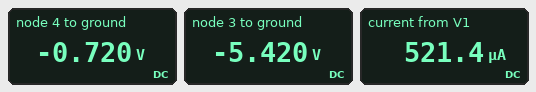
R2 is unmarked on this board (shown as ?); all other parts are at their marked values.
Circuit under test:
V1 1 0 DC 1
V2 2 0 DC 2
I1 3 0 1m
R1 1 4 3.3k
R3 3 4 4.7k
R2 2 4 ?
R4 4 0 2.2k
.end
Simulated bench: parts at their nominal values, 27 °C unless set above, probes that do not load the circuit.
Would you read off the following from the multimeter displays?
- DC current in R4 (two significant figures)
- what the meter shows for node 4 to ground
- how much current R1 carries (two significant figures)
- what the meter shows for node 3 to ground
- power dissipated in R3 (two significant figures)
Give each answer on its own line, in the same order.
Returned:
330 µA
-0.720 V
520 µA
-5.420 V
4.7 mW
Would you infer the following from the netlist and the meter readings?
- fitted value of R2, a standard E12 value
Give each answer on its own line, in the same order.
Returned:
18 kΩ
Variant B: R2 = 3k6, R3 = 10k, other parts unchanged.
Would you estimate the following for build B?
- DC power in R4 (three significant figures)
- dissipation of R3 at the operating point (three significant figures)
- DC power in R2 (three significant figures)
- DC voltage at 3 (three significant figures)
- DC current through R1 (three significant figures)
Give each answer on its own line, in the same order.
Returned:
8.48 µW
10.0 mW
1.27 mW
-10.1 V
344 µA
